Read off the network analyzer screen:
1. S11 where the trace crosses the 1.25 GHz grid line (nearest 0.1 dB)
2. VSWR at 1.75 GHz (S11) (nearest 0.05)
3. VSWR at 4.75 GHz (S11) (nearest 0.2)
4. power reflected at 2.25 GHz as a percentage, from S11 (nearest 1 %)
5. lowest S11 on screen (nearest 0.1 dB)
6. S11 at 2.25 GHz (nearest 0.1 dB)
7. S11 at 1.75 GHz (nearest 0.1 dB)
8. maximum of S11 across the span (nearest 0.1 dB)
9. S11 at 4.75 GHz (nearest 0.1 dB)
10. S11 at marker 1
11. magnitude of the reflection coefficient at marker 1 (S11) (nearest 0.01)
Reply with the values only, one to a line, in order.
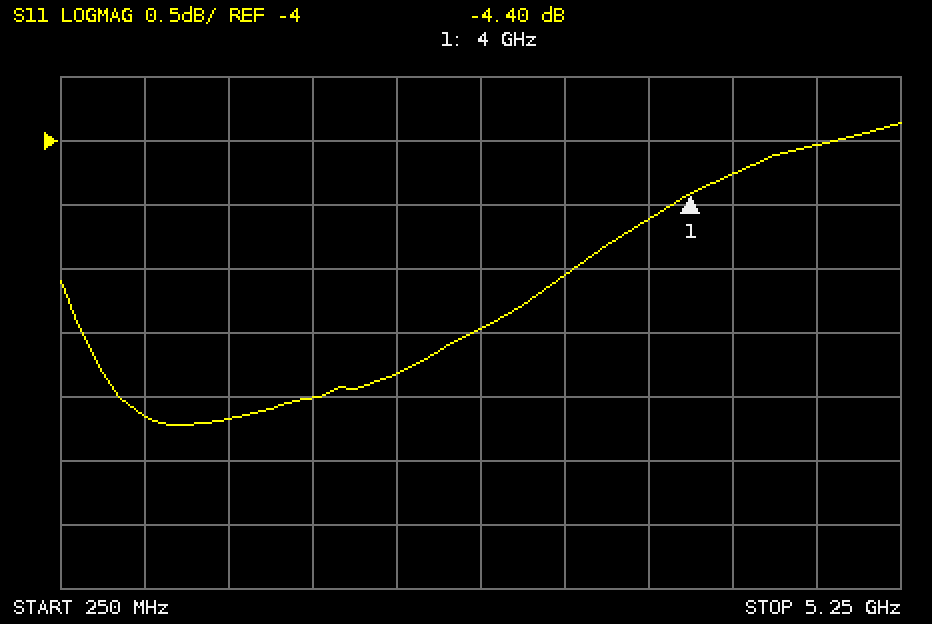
-6.2 dB
3.00
4.4
26 %
-6.2 dB
-5.8 dB
-6.0 dB
-3.9 dB
-4.0 dB
-4.40 dB
0.60
